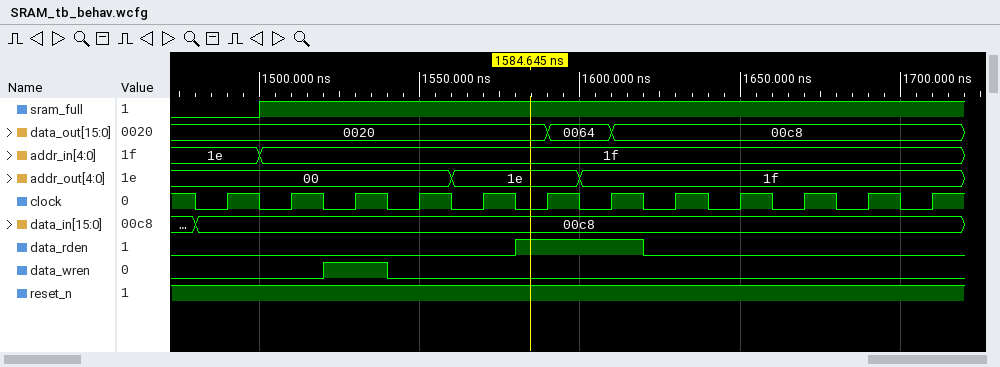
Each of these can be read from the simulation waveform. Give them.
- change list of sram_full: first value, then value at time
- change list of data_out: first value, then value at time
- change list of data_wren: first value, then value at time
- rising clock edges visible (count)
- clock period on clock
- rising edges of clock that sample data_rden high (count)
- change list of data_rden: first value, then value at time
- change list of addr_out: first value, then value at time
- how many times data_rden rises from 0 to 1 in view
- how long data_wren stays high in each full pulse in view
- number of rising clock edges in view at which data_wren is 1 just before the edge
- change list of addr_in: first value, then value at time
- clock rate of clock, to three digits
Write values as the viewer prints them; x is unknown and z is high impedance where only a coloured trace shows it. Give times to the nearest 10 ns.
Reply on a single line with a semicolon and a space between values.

0, 1 at 1500 ns; 0020, 0064 at 1590 ns, 00c8 at 1610 ns; 0, 1 at 1520 ns, 0 at 1540 ns; 12; 20 ns; 2; 0, 1 at 1580 ns, 0 at 1620 ns; 00, 1e at 1560 ns, 1f at 1600 ns; 1; 20 ns; 1; 1e, 1f at 1500 ns; 50.0 MHz
